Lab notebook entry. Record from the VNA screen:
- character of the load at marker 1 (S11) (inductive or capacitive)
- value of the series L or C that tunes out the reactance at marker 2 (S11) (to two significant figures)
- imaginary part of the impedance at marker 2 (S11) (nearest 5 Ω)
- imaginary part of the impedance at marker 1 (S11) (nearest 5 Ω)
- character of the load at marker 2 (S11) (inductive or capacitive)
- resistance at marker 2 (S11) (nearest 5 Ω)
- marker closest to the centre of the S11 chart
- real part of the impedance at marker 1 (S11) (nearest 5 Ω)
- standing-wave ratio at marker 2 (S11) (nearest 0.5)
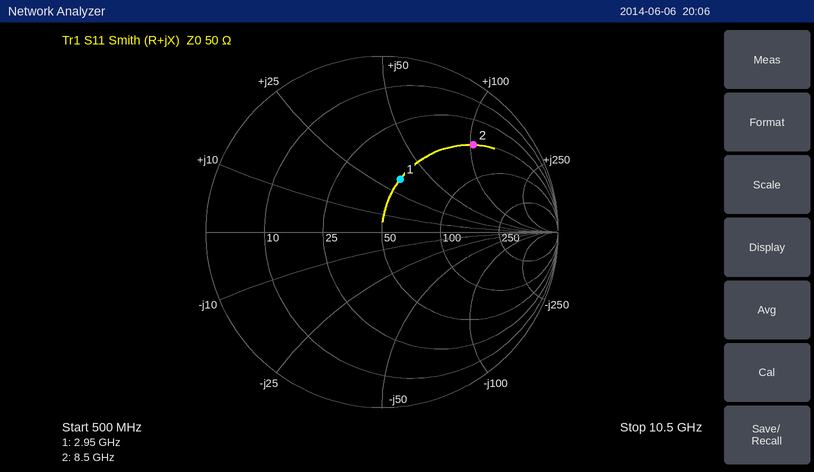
inductive
180 fF
+105 Ω
+35 Ω
inductive
50 Ω
marker 1
50 Ω
6.0
